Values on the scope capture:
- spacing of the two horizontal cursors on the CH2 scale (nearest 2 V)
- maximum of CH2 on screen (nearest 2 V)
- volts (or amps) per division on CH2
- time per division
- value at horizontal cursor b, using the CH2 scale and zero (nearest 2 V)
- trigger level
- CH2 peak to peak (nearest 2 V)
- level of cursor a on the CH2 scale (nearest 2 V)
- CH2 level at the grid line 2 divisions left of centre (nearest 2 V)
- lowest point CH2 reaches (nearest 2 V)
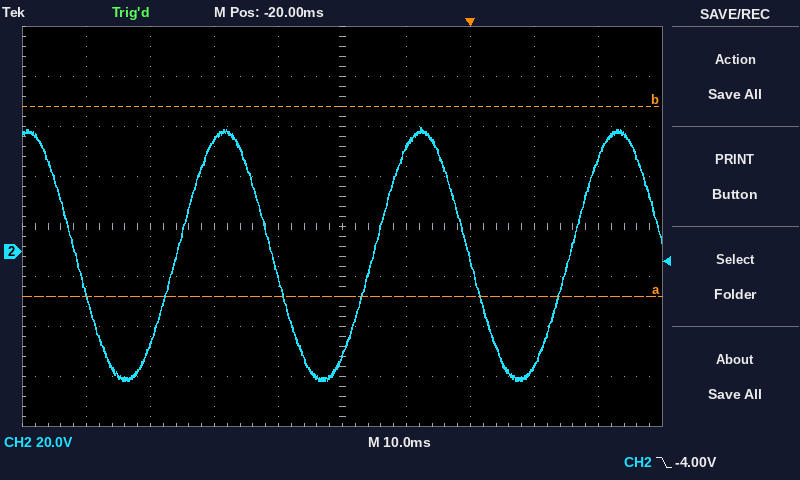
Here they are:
76 V
50 V
20 V
10 ms
58 V
-4.00 V
102 V
-18 V
44 V
-52 V
